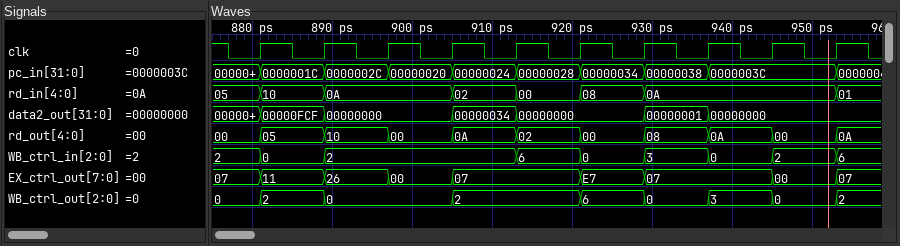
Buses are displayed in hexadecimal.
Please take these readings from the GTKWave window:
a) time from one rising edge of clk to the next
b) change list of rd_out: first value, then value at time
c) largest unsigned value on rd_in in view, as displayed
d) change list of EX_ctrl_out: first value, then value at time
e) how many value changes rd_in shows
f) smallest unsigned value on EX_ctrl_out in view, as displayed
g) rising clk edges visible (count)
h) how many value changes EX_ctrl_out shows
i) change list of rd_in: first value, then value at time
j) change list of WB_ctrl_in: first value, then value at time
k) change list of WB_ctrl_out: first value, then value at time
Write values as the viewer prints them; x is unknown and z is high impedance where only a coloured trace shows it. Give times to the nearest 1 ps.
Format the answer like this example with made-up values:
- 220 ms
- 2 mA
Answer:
- 8 ps
- 00, 05 at 881 ps, 10 at 889 ps, 00 at 897 ps, 0A at 905 ps, 02 at 913 ps, 00 at 921 ps, 08 at 929 ps, 0A at 937 ps, 00 at 945 ps, 0A at 953 ps
- 10
- 07, 11 at 881 ps, 26 at 889 ps, 00 at 897 ps, 07 at 905 ps, E7 at 921 ps, 07 at 929 ps, 00 at 945 ps, 07 at 953 ps
- 7
- 00
- 10
- 8
- 05, 10 at 881 ps, 0A at 889 ps, 02 at 905 ps, 00 at 913 ps, 08 at 921 ps, 0A at 929 ps, 01 at 953 ps
- 2, 0 at 881 ps, 2 at 889 ps, 6 at 913 ps, 0 at 921 ps, 3 at 929 ps, 0 at 937 ps, 2 at 945 ps, 6 at 953 ps
- 0, 2 at 881 ps, 0 at 889 ps, 2 at 905 ps, 6 at 921 ps, 0 at 929 ps, 3 at 937 ps, 0 at 945 ps, 2 at 953 ps
